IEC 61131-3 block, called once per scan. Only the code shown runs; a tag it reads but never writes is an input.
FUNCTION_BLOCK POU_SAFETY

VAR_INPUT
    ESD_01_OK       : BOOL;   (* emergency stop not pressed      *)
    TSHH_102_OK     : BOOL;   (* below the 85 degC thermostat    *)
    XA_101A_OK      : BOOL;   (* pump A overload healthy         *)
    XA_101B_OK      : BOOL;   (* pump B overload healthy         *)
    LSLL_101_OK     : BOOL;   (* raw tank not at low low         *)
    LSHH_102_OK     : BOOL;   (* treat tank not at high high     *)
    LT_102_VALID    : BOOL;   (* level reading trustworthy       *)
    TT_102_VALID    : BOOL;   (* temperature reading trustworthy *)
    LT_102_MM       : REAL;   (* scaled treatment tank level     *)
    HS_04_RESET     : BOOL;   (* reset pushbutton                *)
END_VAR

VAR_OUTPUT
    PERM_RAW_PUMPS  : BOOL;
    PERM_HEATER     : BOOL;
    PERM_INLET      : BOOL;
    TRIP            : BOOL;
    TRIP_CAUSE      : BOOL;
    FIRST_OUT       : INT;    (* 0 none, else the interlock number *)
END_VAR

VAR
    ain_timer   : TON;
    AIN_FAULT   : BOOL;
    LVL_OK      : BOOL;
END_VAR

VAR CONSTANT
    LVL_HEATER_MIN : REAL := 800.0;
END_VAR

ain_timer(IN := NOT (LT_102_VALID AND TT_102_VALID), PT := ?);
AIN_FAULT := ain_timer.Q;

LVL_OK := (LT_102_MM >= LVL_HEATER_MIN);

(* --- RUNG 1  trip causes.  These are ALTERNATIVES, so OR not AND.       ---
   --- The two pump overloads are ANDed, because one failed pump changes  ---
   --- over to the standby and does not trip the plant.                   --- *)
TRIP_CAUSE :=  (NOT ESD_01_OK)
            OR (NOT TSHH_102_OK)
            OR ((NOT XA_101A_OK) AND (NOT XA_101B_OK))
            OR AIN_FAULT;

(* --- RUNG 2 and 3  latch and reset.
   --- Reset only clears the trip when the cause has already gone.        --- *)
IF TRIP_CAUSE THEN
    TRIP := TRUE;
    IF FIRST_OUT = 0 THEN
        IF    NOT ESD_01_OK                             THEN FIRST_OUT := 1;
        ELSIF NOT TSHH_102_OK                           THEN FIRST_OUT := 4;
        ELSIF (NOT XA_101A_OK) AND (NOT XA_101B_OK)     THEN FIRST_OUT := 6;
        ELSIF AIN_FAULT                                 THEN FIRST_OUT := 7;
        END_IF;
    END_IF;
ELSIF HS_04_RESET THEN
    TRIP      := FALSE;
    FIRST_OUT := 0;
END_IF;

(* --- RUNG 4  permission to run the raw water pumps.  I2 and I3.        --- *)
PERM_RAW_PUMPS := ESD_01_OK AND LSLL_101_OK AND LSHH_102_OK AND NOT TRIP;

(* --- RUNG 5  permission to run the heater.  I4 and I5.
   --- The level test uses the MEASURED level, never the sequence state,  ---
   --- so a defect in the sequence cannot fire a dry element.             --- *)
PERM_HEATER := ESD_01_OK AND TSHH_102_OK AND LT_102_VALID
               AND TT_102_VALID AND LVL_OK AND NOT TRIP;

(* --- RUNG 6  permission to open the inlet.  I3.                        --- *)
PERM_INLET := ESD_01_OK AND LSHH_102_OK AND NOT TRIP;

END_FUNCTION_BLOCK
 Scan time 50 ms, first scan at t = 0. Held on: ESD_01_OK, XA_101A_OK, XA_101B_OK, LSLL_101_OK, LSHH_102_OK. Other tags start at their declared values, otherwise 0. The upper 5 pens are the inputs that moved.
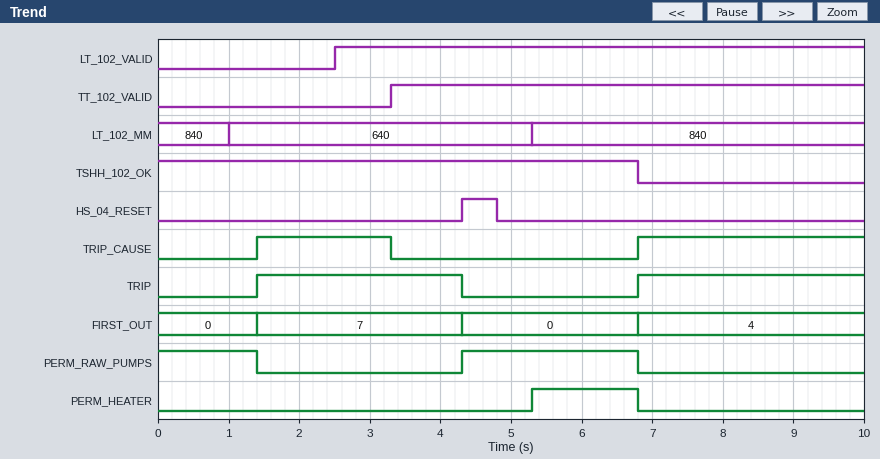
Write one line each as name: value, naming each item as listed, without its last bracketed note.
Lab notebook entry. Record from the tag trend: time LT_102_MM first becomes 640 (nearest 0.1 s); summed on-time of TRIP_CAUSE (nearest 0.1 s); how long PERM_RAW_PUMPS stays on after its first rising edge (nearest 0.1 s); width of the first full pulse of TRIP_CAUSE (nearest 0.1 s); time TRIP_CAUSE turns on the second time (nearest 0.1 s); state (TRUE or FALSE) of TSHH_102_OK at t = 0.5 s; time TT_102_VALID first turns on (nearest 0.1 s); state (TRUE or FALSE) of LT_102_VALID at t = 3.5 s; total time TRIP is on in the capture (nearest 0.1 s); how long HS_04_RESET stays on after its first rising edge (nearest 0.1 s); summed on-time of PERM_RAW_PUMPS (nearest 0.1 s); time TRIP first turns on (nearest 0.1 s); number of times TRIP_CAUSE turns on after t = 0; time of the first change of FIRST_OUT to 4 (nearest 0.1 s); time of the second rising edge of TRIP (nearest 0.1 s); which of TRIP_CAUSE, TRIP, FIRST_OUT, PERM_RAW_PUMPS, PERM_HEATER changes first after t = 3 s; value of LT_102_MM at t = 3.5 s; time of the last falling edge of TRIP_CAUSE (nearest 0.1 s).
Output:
time LT_102_MM first becomes 640: 1.0 s
summed on-time of TRIP_CAUSE: 5.1 s
how long PERM_RAW_PUMPS stays on after its first rising edge: 2.5 s
width of the first full pulse of TRIP_CAUSE: 1.9 s
time TRIP_CAUSE turns on the second time: 6.8 s
state (TRUE or FALSE) of TSHH_102_OK at t = 0.5 s: TRUE
time TT_102_VALID first turns on: 3.3 s
state (TRUE or FALSE) of LT_102_VALID at t = 3.5 s: TRUE
total time TRIP is on in the capture: 6.1 s
how long HS_04_RESET stays on after its first rising edge: 0.5 s
summed on-time of PERM_RAW_PUMPS: 3.9 s
time TRIP first turns on: 1.4 s
number of times TRIP_CAUSE turns on after t = 0: 2
time of the first change of FIRST_OUT to 4: 6.8 s
time of the second rising edge of TRIP: 6.8 s
which of TRIP_CAUSE, TRIP, FIRST_OUT, PERM_RAW_PUMPS, PERM_HEATER changes first after t = 3 s: TRIP_CAUSE
value of LT_102_MM at t = 3.5 s: 640
time of the last falling edge of TRIP_CAUSE: 3.3 s
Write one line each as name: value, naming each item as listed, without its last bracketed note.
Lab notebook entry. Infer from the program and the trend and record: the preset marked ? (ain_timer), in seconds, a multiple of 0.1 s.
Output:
the preset marked ? (ain_timer), in seconds, a multiple of 0.1 s: 1.4 s
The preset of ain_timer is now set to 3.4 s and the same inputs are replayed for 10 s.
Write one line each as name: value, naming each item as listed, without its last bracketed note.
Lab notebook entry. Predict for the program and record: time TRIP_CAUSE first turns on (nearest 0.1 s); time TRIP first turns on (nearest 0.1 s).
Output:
time TRIP_CAUSE first turns on: 6.8 s
time TRIP first turns on: 6.8 s
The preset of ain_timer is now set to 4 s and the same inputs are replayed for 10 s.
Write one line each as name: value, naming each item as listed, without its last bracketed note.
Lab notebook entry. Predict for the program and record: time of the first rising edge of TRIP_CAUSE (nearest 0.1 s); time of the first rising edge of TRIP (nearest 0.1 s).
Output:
time of the first rising edge of TRIP_CAUSE: 6.8 s
time of the first rising edge of TRIP: 6.8 s
